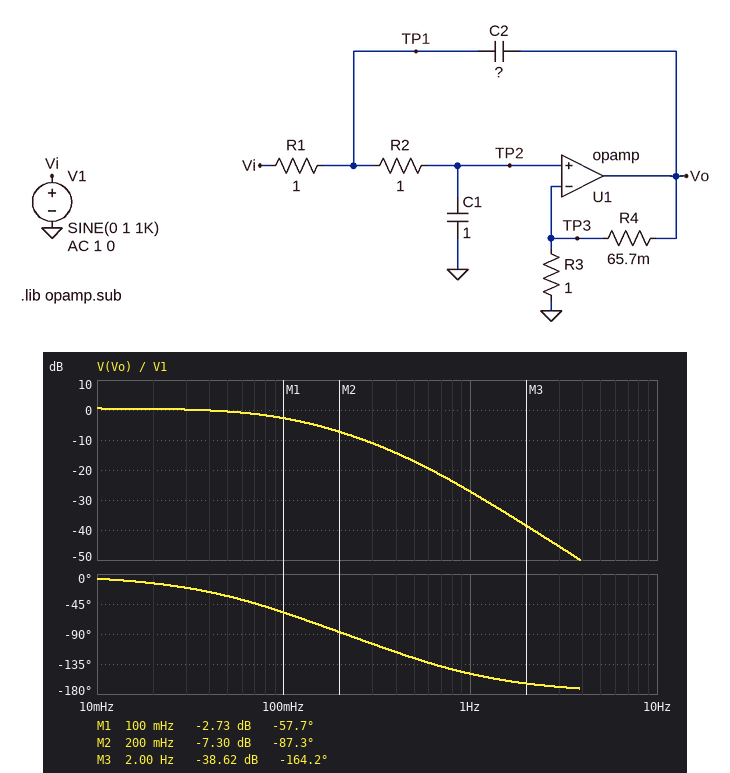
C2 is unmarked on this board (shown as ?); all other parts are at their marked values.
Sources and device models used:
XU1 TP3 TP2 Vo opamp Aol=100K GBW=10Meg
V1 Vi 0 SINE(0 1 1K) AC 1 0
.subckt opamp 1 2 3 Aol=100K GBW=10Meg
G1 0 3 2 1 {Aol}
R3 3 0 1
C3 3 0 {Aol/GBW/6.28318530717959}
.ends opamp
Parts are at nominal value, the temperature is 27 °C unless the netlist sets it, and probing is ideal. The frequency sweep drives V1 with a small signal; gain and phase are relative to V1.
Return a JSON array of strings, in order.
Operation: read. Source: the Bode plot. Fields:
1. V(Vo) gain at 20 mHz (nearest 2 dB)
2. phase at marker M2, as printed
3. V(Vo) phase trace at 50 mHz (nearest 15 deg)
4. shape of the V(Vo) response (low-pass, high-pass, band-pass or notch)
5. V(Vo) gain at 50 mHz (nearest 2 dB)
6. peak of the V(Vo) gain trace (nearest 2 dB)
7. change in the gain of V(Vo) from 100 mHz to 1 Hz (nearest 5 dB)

["0 dB", "-87.3 deg", "-30 deg", "low-pass", "0 dB", "0 dB", "-25 dB"]
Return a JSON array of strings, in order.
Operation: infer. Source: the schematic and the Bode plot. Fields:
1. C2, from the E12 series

["560 mF"]
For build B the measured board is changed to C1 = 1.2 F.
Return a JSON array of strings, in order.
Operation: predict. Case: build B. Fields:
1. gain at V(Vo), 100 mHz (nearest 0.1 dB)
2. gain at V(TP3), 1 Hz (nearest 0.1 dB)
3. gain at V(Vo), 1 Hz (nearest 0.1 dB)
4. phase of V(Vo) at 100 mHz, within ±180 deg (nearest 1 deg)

["-3.8 dB", "-29.4 dB", "-28.9 dB", "-64 deg"]
